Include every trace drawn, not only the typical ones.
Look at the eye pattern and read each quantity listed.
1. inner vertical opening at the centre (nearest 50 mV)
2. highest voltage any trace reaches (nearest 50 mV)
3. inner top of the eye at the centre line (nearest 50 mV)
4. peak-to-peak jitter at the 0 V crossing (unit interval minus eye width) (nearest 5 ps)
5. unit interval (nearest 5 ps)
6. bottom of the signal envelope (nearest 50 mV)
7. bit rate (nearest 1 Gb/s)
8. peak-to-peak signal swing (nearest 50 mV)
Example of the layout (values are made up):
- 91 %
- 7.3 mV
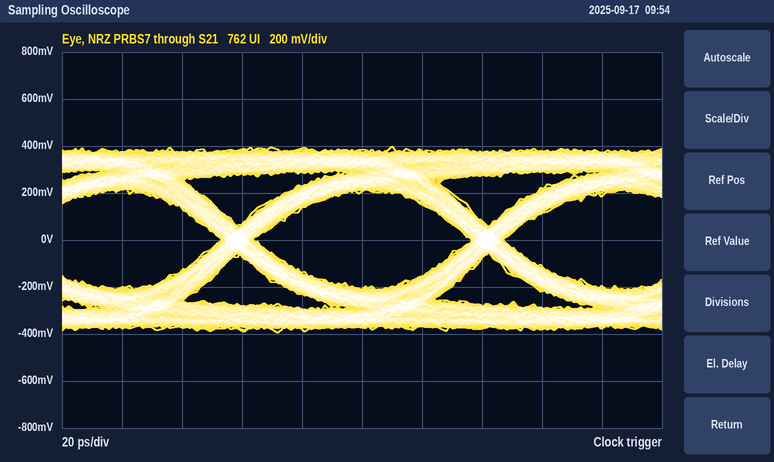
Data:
- 400 mV
- 400 mV
- 200 mV
- 10 ps
- 85 ps
- -400 mV
- 12 Gb/s
- 800 mV
